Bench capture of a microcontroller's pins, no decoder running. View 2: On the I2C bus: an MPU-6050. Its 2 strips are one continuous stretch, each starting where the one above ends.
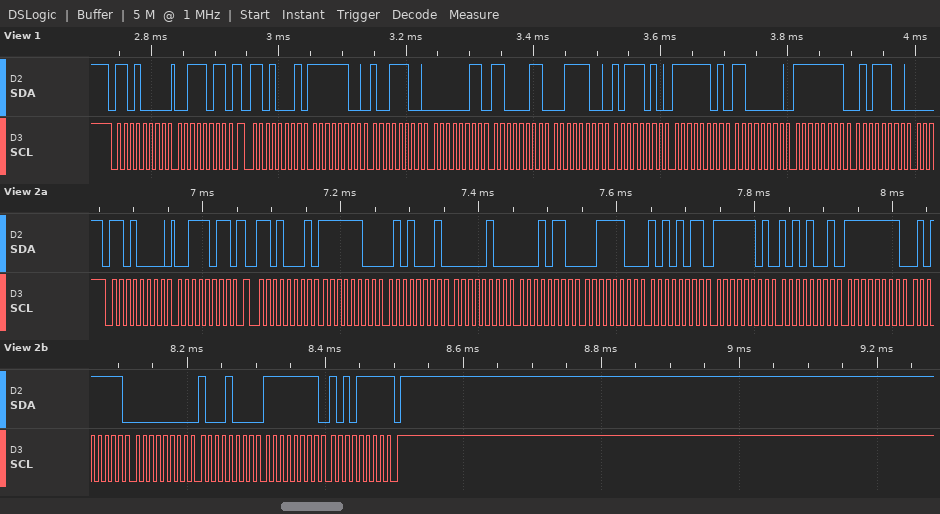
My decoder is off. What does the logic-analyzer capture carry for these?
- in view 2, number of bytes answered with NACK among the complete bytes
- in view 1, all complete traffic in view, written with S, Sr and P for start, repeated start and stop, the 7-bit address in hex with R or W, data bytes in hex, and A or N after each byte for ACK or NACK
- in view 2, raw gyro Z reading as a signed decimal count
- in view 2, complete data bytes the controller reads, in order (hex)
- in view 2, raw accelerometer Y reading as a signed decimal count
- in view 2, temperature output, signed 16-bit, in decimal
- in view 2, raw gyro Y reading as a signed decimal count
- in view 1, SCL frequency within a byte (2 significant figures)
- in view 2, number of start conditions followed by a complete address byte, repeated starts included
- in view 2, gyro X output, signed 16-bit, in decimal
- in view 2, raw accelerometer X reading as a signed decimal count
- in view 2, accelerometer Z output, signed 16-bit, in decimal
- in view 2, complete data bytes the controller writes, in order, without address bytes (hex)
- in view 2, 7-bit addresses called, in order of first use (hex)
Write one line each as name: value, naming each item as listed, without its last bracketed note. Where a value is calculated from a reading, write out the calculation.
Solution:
in view 2, number of bytes answered with NACK among the complete bytes: 1
in view 1, all complete traffic in view, written with S, Sr and P for start, repeated start and stop, the 7-bit address in hex with R or W, data bytes in hex, and A or N after each byte for ACK or NACK: S 68W A 3B A Sr 68R A FC A 9C A 03 A C3 A 3C A BA A FD A C0 A FF A 5C A
in view 2, raw gyro Z reading as a signed decimal count: 0xFFAF = -81
in view 2, complete data bytes the controller reads, in order: FC 51 04 16 3C AB FD A9 FF 5F 00 88 FF AF
in view 2, raw accelerometer Y reading as a signed decimal count: 0x0416 = 1046
in view 2, temperature output, signed 16-bit, in decimal: 0xFDA9 = -599
in view 2, raw gyro Y reading as a signed decimal count: 0x0088 = 136
in view 1, SCL frequency within a byte: 100 kHz
in view 2, number of start conditions followed by a complete address byte, repeated starts included: 2
in view 2, gyro X output, signed 16-bit, in decimal: 0xFF5F = -161
in view 2, raw accelerometer X reading as a signed decimal count: 0xFC51 = -943
in view 2, accelerometer Z output, signed 16-bit, in decimal: 0x3CAB = 15531
in view 2, complete data bytes the controller writes, in order, without address bytes: 3B
in view 2, 7-bit addresses called, in order of first use: 0x68
